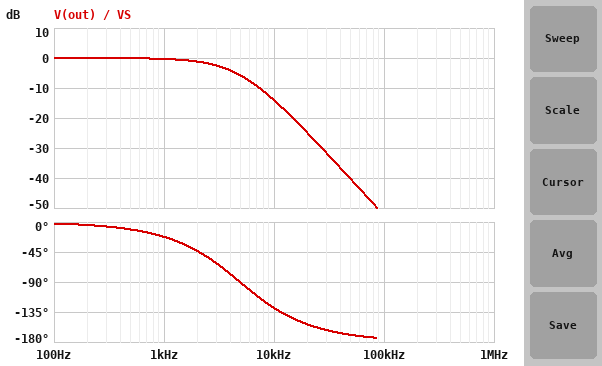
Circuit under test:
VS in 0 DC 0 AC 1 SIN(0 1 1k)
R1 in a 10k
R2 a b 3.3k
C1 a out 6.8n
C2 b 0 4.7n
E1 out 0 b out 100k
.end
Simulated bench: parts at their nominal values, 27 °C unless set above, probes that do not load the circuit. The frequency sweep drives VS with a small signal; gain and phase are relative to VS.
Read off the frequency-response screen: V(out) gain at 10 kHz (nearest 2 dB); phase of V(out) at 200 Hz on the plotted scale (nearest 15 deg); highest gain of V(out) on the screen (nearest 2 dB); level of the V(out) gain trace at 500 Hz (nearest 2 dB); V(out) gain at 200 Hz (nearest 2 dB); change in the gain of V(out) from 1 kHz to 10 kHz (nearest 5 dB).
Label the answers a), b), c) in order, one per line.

a) -14 dB
b) 0 deg
c) 0 dB
d) 0 dB
e) 0 dB
f) -15 dB
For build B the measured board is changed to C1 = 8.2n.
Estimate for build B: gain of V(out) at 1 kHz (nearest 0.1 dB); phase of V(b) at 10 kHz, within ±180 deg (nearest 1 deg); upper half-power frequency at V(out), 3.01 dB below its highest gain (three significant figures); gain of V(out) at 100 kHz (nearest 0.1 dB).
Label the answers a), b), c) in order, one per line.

a) -0.2 dB
b) -136 deg
c) 3.45 kHz
d) -54.0 dB
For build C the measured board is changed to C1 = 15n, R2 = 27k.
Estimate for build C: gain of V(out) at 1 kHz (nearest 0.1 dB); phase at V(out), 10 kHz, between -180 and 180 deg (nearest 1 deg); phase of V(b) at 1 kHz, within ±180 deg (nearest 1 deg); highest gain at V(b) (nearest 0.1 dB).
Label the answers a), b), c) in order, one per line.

a) -1.0 dB
b) -172 deg
c) -77 deg
d) 0.2 dB
